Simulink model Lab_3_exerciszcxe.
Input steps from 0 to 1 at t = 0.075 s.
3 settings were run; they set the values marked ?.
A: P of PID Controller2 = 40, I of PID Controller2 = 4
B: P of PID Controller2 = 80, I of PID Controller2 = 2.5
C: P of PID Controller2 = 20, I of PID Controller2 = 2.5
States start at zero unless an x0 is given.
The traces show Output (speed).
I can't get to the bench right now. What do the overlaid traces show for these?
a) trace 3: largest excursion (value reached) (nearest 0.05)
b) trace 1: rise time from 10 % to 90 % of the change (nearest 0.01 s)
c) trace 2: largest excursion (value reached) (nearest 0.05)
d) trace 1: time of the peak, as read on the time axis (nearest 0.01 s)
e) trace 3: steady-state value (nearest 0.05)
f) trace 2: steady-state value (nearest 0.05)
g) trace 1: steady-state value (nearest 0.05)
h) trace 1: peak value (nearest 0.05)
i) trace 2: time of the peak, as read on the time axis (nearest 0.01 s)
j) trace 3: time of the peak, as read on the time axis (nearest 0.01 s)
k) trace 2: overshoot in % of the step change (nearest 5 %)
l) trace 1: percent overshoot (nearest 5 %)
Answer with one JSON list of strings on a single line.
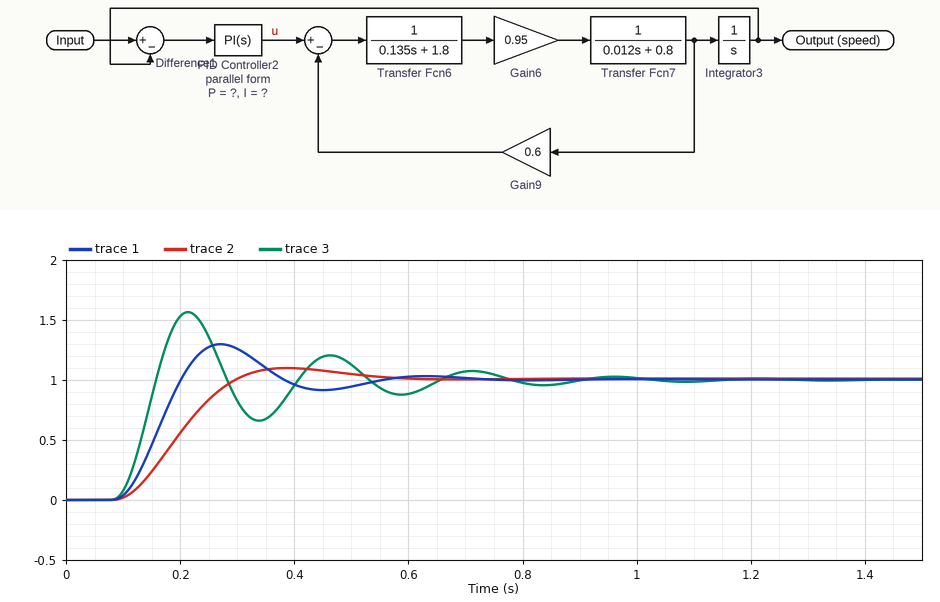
["1.55", "0.08 s", "1.10", "0.27 s", "1.00", "1.00", "1.00", "1.30", "0.39 s", "0.21 s", "10 %", "30 %"]
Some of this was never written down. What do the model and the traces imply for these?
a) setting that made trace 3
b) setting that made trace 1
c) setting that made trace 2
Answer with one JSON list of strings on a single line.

["B", "A", "C"]
